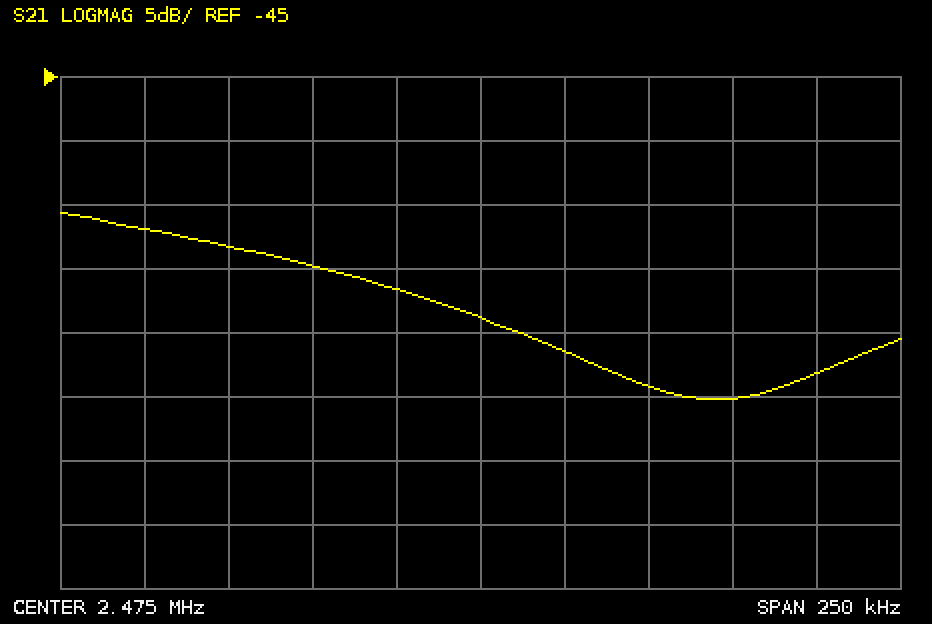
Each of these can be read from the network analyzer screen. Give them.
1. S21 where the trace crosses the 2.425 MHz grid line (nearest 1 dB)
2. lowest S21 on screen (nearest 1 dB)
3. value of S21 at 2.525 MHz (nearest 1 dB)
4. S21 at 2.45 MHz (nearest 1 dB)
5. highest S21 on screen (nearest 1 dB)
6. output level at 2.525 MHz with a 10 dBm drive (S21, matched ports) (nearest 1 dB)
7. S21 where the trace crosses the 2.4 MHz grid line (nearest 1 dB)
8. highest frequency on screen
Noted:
-60 dB
-70 dB
-69 dB
-62 dB
-56 dB
-59 dBm
-58 dB
2.6 MHz
